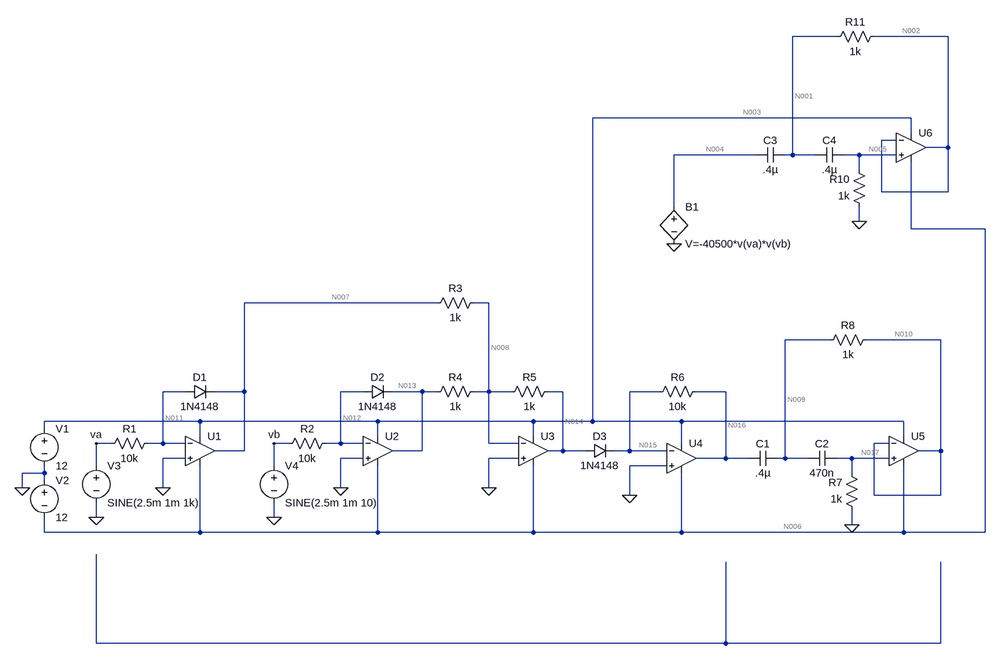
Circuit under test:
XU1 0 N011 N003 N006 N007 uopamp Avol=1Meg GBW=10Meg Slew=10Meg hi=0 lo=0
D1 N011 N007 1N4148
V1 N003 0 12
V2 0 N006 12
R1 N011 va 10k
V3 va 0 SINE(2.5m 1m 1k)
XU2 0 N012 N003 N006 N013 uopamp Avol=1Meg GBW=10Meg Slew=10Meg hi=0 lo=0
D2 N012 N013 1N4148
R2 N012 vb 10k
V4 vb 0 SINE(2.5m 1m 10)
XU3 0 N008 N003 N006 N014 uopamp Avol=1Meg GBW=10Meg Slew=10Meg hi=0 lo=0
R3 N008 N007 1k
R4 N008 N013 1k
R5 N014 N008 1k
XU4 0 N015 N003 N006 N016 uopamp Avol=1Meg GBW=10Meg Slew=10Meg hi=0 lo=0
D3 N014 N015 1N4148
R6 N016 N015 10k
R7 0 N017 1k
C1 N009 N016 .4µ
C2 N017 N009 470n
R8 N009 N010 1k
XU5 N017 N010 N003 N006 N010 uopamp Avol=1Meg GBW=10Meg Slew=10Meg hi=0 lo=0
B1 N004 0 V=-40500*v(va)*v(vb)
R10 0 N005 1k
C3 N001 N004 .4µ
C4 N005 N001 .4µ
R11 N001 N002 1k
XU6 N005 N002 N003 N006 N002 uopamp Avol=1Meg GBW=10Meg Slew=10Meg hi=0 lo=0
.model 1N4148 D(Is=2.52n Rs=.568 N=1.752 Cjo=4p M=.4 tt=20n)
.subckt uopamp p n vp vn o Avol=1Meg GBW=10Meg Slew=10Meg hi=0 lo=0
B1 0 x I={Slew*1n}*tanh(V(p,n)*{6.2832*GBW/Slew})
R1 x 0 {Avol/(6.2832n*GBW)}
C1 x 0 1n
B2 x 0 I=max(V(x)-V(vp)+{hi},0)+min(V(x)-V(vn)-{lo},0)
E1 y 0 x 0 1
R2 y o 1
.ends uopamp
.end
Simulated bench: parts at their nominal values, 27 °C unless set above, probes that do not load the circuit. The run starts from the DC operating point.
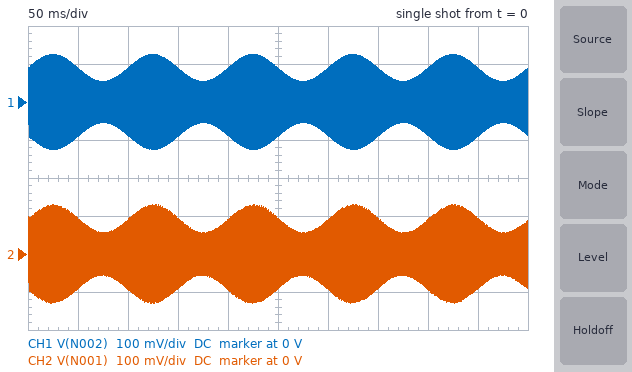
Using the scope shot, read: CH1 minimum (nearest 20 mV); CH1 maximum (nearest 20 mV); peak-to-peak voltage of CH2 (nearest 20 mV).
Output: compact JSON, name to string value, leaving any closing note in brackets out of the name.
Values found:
{"CH1 minimum": "-120 mV", "CH1 maximum": "120 mV", "peak-to-peak voltage of CH2": "260 mV"}
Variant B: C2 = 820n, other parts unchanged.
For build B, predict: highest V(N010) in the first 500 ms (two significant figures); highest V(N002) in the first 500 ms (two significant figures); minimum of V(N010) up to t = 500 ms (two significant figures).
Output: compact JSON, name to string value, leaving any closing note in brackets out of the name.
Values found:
{"highest V(N010) in the first 500 ms": "130 mV", "highest V(N002) in the first 500 ms": "120 mV", "minimum of V(N010) up to t = 500 ms": "-130 mV"}
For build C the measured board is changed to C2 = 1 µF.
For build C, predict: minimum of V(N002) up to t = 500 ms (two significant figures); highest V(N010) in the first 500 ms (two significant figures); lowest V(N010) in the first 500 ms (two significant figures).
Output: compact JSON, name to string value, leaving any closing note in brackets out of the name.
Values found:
{"minimum of V(N002) up to t = 500 ms": "-120 mV", "highest V(N010) in the first 500 ms": "130 mV", "lowest V(N010) in the first 500 ms": "-130 mV"}
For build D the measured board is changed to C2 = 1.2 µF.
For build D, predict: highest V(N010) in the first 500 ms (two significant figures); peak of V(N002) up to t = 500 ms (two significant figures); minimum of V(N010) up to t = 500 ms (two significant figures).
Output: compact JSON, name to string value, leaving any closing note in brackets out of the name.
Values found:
{"highest V(N010) in the first 500 ms": "130 mV", "peak of V(N002) up to t = 500 ms": "120 mV", "minimum of V(N010) up to t = 500 ms": "-130 mV"}
